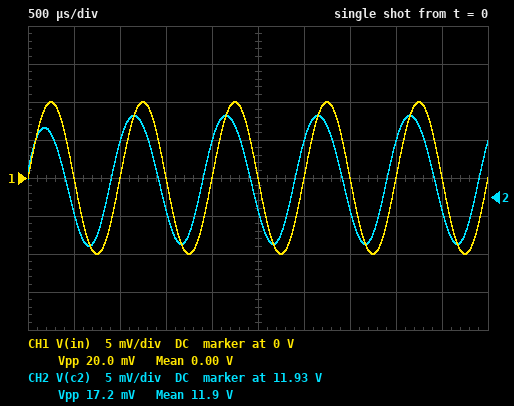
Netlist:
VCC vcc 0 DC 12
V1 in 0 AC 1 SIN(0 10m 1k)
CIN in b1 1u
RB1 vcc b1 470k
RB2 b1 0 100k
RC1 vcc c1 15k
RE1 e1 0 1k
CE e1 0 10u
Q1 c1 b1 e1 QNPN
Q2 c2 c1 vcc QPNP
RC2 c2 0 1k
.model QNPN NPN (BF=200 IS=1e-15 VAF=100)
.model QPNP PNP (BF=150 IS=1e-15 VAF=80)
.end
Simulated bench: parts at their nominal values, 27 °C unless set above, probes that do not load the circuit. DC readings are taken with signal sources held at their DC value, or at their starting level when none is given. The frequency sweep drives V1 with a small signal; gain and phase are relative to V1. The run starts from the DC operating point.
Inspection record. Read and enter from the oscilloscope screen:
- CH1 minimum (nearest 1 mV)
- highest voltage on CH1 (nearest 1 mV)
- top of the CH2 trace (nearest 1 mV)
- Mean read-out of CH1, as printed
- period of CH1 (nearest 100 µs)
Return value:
-10 mV
10 mV
11.936 V
0.00 V
1.0 ms
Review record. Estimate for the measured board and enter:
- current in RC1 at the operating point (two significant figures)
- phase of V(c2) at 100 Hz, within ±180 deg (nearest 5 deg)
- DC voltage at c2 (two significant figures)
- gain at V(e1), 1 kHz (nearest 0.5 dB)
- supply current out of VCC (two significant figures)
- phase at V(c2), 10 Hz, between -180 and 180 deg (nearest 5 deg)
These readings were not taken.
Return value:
52 µA
75 deg
12 V
-5.5 dB
13 mA
45 deg
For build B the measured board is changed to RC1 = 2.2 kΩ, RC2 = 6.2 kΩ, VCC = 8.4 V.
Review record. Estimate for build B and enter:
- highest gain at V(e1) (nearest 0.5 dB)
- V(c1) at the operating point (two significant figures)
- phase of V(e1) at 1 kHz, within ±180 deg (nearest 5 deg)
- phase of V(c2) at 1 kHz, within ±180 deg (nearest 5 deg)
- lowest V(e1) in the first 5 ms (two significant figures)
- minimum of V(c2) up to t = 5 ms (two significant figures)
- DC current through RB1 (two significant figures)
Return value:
-1.0 dB
7.7 V
-70 deg
20 deg
560 mV
8.3 V
15 µA
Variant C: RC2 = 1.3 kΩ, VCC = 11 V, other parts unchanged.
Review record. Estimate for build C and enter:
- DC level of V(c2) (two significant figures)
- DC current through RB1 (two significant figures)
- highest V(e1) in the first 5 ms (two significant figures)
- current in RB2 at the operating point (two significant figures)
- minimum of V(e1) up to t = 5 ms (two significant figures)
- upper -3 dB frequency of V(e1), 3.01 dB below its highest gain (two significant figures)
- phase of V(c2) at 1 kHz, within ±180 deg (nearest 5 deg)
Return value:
11 V
20 µA
890 mV
16 µA
880 mV
590 Hz
30 deg
